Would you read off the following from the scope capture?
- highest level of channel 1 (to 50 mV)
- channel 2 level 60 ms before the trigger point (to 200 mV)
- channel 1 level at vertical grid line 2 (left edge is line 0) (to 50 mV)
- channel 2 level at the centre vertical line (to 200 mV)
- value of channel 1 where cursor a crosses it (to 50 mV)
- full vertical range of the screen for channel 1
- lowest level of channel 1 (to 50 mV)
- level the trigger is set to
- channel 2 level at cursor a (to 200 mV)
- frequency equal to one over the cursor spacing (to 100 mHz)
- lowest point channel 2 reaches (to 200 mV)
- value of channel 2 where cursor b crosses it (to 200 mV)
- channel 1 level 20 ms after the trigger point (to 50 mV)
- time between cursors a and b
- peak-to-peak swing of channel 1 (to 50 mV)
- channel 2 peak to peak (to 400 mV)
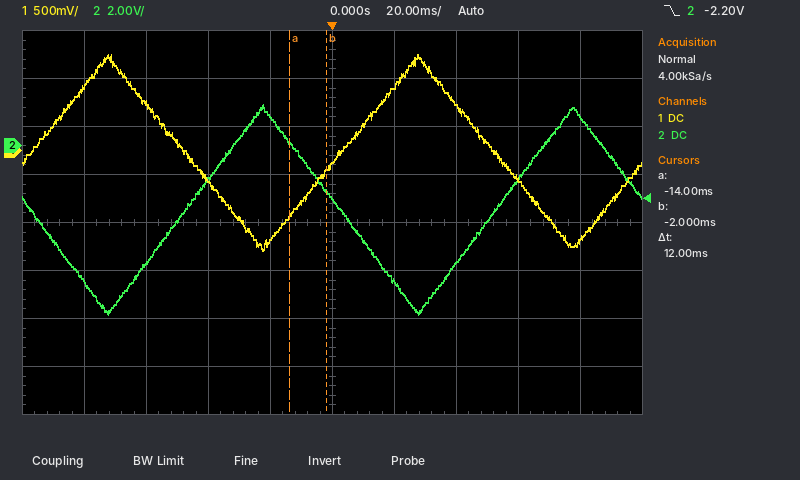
1.00 V
-4.8 V
500 mV
-2.2 V
-700 mV
4 V
-1.05 V
-2.20 V
200 mV
83.3 Hz
-7.0 V
-2.0 V
700 mV
12 ms
2.05 V
8.8 V
